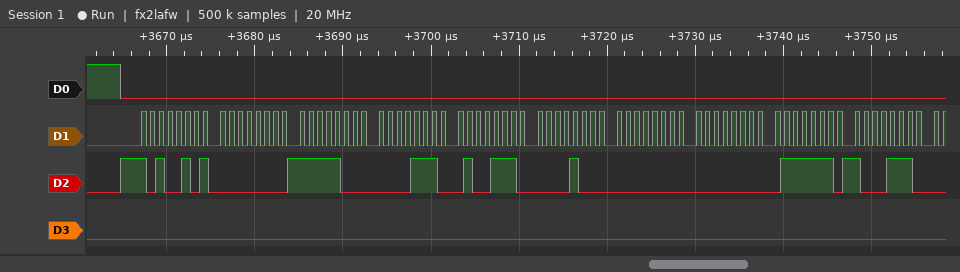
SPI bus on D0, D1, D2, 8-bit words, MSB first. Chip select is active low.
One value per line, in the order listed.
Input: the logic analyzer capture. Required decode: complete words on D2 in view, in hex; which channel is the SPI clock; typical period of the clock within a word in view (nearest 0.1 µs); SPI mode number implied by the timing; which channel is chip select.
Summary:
A5, 00, F8, 0E, 4E, 08, 00, 00, 7E, 8E
D1
1 µs
0
D0
